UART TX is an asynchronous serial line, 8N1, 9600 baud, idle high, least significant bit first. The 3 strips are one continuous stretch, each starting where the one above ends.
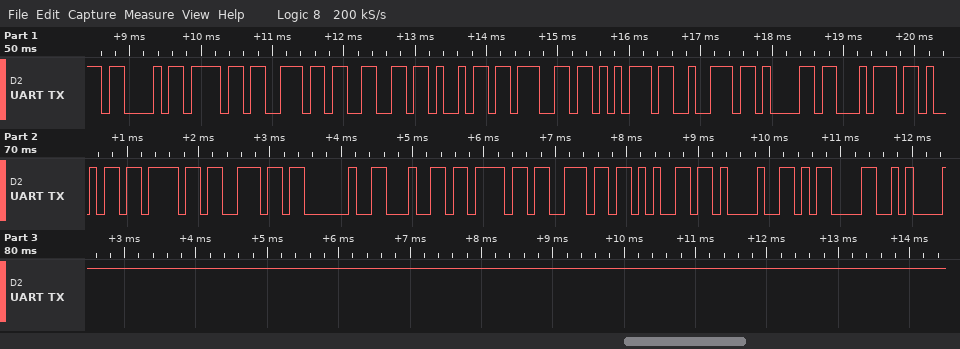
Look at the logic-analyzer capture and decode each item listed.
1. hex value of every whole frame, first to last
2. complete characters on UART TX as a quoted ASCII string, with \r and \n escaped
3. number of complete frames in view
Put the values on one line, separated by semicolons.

43 6F 6E 66 69 67 75 72 61 74 69 6F 6E 20 64 6F 6E 65 21 0D 0A; "Configuration done!\r\n"; 21
